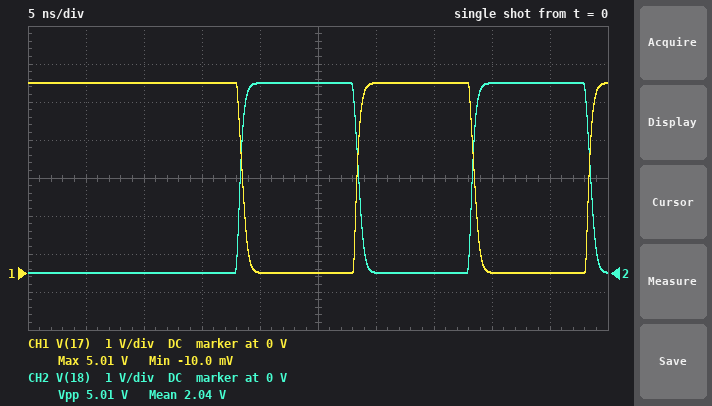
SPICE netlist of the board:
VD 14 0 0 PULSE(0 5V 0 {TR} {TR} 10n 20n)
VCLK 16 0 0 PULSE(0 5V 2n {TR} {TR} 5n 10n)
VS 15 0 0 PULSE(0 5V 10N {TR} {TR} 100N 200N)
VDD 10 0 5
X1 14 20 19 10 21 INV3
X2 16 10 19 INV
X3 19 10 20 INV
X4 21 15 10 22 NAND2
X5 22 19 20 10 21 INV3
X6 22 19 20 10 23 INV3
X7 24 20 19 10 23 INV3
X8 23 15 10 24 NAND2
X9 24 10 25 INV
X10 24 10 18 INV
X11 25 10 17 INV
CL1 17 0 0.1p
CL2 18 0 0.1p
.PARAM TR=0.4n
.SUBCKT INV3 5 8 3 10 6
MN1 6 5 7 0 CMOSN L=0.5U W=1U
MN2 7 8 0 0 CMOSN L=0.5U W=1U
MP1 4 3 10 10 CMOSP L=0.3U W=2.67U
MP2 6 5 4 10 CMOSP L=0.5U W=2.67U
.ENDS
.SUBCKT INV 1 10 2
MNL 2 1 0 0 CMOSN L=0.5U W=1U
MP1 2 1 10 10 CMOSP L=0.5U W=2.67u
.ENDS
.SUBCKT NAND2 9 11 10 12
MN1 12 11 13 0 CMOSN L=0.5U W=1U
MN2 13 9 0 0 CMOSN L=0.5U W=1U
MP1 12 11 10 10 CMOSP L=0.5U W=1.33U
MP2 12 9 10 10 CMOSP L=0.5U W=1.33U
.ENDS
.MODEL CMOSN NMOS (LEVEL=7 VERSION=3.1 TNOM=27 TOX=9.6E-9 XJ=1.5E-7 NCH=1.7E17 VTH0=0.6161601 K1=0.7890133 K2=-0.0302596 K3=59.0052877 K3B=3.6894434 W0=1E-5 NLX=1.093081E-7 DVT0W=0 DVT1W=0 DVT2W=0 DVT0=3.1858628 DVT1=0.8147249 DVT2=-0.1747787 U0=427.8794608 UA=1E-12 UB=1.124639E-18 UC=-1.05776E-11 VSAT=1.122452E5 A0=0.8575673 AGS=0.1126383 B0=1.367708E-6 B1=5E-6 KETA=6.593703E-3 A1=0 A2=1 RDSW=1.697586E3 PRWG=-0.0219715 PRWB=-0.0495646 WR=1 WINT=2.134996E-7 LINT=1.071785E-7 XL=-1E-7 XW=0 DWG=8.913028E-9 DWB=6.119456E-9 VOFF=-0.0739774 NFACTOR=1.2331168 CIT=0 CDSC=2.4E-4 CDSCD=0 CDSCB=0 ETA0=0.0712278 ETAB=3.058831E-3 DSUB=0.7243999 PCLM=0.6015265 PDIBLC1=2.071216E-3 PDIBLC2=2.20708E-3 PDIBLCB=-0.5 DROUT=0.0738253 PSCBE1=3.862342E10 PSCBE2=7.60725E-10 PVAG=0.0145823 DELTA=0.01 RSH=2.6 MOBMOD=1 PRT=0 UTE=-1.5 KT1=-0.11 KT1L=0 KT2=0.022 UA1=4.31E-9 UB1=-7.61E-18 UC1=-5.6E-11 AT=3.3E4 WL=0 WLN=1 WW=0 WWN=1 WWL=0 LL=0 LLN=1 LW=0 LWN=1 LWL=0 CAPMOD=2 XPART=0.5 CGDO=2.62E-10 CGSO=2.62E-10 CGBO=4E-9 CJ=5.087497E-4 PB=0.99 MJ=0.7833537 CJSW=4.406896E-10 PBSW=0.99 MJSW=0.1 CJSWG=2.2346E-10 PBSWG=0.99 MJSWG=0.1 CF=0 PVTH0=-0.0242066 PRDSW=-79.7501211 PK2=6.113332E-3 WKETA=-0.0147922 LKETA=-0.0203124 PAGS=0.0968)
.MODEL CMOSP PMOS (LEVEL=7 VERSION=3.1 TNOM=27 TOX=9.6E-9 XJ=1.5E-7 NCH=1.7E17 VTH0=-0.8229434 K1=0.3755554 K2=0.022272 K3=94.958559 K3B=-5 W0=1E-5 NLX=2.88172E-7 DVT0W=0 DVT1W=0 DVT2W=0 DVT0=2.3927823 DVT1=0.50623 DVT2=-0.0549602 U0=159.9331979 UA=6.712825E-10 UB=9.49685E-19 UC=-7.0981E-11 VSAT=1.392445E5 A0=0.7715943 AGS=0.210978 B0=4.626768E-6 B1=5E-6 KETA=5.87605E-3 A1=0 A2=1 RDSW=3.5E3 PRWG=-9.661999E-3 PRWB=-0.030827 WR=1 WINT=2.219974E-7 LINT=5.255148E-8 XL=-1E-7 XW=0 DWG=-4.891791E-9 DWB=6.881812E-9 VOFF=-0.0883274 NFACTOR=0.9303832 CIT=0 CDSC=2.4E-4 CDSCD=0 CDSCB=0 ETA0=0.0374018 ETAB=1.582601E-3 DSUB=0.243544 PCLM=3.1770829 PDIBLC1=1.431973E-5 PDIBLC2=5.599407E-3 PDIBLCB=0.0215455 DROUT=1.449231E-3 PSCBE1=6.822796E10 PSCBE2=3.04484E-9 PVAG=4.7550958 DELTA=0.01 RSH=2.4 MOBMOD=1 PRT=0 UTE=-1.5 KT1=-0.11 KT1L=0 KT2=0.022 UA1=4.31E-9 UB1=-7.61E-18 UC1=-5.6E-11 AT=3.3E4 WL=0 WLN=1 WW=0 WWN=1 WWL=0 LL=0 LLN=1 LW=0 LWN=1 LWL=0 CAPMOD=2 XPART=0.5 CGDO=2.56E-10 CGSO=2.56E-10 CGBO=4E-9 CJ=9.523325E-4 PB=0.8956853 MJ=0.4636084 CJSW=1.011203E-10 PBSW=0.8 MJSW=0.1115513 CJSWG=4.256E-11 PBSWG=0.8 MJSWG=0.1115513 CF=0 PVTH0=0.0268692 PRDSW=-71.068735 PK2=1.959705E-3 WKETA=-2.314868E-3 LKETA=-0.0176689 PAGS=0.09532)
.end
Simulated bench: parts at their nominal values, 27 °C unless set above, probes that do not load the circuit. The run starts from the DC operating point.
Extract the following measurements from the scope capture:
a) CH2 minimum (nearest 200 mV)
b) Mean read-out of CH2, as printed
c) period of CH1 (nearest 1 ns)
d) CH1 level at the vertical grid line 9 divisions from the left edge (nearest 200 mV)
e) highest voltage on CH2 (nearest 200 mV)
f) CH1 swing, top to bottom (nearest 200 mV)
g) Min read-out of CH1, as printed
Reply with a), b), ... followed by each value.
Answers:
a) 0 V
b) 2.04 V
c) 20 ns
d) 0 V
e) 5.0 V
f) 5.0 V
g) -10.0 mV
